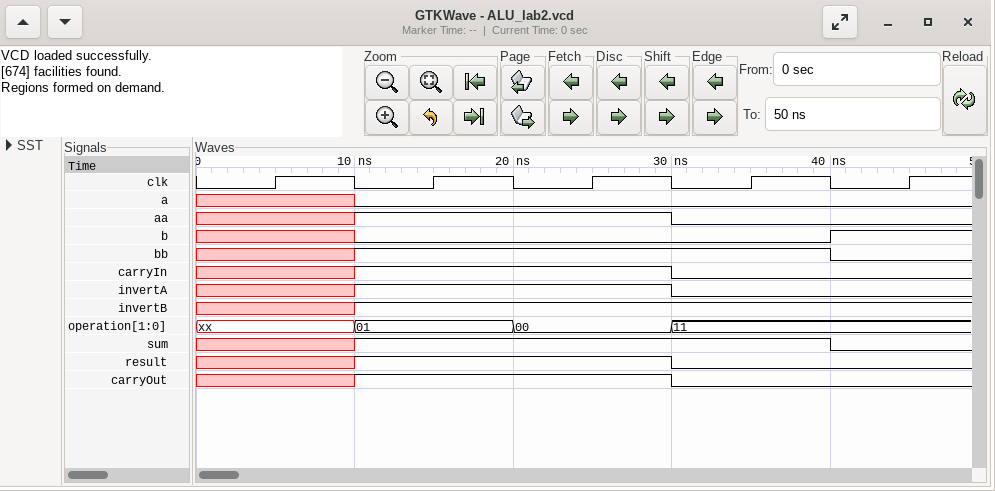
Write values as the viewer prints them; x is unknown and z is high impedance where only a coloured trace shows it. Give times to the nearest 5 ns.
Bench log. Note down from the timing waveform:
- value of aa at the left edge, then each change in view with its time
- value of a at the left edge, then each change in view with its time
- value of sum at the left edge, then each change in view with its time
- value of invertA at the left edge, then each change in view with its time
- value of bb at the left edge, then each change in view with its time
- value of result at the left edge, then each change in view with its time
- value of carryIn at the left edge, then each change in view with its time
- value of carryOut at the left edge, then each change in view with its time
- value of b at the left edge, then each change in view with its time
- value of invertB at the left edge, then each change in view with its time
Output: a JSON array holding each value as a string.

["x, 1 at 10 ns, 0 at 30 ns", "x, 0 at 10 ns", "x, 1 at 10 ns, 0 at 40 ns", "x, 1 at 10 ns, 0 at 30 ns", "x, 1 at 10 ns, 0 at 40 ns", "x, 1 at 10 ns, 0 at 30 ns", "x, 1 at 10 ns, 0 at 30 ns", "x, 1 at 10 ns, 0 at 30 ns", "x, 0 at 10 ns, 1 at 40 ns", "x, 1 at 10 ns"]
